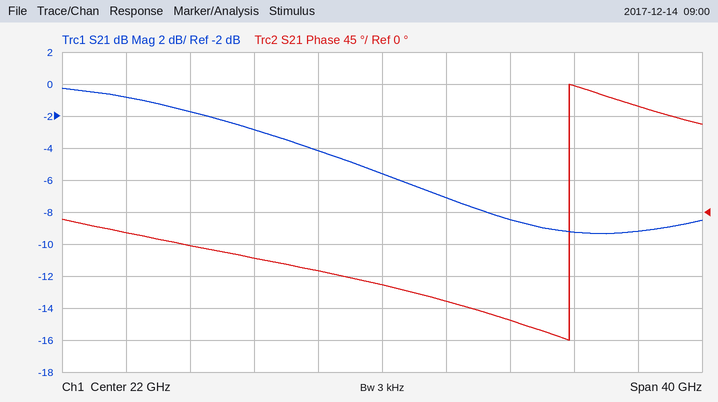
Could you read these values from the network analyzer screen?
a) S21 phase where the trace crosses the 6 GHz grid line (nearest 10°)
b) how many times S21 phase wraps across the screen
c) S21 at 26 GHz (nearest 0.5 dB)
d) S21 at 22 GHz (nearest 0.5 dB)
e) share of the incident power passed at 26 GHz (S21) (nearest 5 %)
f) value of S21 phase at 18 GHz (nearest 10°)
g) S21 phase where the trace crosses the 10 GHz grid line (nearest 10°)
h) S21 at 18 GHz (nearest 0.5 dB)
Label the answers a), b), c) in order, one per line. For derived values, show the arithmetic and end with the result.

a) -30°
b) 1
c) -7.0 dB
d) -5.5 dB
e) 10^(-7/10) ≈ 20 %
f) -80°
g) -50°
h) -4.0 dB
